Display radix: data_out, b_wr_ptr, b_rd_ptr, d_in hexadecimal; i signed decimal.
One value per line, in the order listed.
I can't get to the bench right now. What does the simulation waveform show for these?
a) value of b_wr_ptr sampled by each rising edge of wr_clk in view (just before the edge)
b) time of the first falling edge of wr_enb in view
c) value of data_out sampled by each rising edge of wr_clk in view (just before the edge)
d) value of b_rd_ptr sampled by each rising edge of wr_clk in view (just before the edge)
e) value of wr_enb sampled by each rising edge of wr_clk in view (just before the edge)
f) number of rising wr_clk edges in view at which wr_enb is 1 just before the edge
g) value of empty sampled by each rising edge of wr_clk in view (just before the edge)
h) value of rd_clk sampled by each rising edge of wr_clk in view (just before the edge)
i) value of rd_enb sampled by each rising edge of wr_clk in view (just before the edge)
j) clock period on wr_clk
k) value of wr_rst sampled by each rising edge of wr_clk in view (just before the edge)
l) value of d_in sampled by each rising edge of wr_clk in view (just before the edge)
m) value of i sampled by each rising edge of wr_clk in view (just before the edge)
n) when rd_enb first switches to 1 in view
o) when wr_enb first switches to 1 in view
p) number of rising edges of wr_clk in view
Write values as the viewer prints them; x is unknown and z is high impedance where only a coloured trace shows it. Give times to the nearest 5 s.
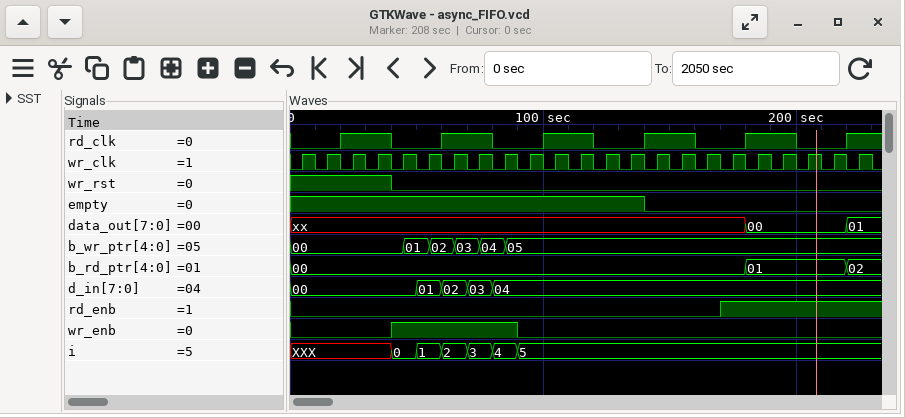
00, 00, 00, 00, 00, 01, 02, 03, 04, 05, 05, 05, 05, 05, 05, 05, 05, 05, 05, 05, 05, 05, 05
90 s
xx, xx, xx, xx, xx, xx, xx, xx, xx, xx, xx, xx, xx, xx, xx, xx, xx, xx, 00, 00, 00, 00, 01
00, 00, 00, 00, 00, 00, 00, 00, 00, 00, 00, 00, 00, 00, 00, 00, 00, 00, 01, 01, 01, 01, 02
0 0 0 0 1 1 1 1 1 0 0 0 0 0 0 0 0 0 0 0 0 0 0
5
1 1 1 1 1 1 1 1 1 1 1 1 1 1 0 0 0 0 0 0 0 0 0
0 0 1 1 0 0 1 1 0 0 1 1 0 0 1 1 0 0 1 1 0 0 1
0 0 0 0 0 0 0 0 0 0 0 0 0 0 0 0 0 1 1 1 1 1 1
10 s
1 1 1 1 0 0 0 0 0 0 0 0 0 0 0 0 0 0 0 0 0 0 0
00, 00, 00, 00, 00, 01, 02, 03, 04, 04, 04, 04, 04, 04, 04, 04, 04, 04, 04, 04, 04, 04, 04
XXX, XXX, XXX, XXX, 0, 1, 2, 3, 4, 5, 5, 5, 5, 5, 5, 5, 5, 5, 5, 5, 5, 5, 5
170 s
40 s
23
